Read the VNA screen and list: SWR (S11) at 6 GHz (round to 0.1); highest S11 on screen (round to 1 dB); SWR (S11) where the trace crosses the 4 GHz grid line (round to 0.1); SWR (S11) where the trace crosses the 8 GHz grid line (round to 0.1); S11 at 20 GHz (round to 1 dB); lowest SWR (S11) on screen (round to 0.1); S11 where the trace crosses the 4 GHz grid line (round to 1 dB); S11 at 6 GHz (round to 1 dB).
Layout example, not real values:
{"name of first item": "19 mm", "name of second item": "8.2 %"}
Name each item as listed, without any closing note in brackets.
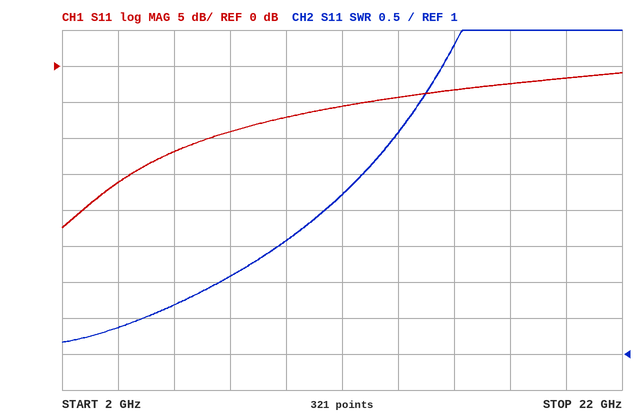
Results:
{"SWR (S11) at 6 GHz": "1.7", "highest S11 on screen": "-1 dB", "SWR (S11) where the trace crosses the 4 GHz grid line": "1.4", "SWR (S11) where the trace crosses the 8 GHz grid line": "2.1", "S11 at 20 GHz": "-2 dB", "lowest SWR (S11) on screen": "1.2", "S11 where the trace crosses the 4 GHz grid line": "-16 dB", "S11 at 6 GHz": "-12 dB"}
